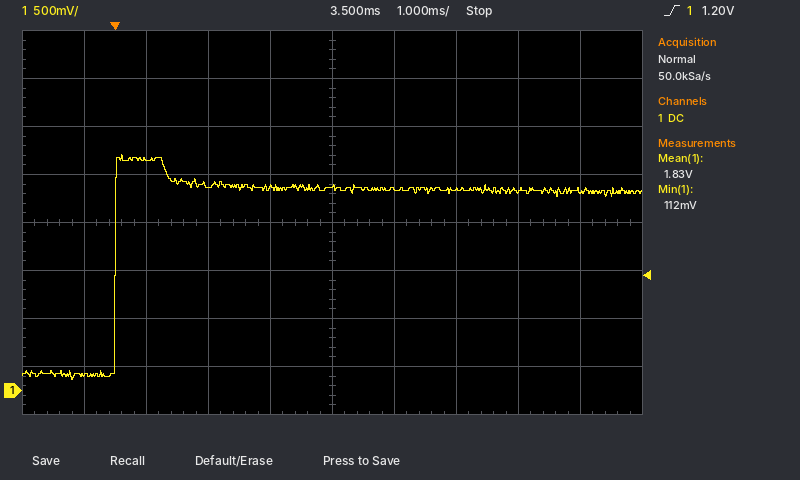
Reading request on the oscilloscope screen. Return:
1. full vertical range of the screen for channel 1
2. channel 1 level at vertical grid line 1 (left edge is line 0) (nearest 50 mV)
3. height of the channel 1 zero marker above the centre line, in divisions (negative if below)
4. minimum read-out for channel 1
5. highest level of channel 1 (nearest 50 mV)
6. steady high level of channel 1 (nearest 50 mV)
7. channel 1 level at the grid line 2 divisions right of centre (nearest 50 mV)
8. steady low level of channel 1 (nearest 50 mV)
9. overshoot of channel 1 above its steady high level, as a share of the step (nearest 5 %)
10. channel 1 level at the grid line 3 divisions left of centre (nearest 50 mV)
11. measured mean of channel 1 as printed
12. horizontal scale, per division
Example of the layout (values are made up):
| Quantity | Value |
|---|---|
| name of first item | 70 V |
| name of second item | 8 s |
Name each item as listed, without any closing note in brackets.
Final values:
| Quantity | Value |
|---|---|
| full vertical range of the screen for channel 1 | 4 V |
| channel 1 level at vertical grid line 1 (left edge is line 0) | 150 mV |
| height of the channel 1 zero marker above the centre line, in divisions | -3.5 div |
| minimum read-out for channel 1 | 112 mV |
| highest level of channel 1 | 2.45 V |
| steady high level of channel 1 | 2.10 V |
| channel 1 level at the grid line 2 divisions right of centre | 2.10 V |
| steady low level of channel 1 | 150 mV |
| overshoot of channel 1 above its steady high level, as a share of the step | 20 % |
| channel 1 level at the grid line 3 divisions left of centre | 2.40 V |
| measured mean of channel 1 as printed | 1.83 V |
| horizontal scale, per division | 1 ms |
